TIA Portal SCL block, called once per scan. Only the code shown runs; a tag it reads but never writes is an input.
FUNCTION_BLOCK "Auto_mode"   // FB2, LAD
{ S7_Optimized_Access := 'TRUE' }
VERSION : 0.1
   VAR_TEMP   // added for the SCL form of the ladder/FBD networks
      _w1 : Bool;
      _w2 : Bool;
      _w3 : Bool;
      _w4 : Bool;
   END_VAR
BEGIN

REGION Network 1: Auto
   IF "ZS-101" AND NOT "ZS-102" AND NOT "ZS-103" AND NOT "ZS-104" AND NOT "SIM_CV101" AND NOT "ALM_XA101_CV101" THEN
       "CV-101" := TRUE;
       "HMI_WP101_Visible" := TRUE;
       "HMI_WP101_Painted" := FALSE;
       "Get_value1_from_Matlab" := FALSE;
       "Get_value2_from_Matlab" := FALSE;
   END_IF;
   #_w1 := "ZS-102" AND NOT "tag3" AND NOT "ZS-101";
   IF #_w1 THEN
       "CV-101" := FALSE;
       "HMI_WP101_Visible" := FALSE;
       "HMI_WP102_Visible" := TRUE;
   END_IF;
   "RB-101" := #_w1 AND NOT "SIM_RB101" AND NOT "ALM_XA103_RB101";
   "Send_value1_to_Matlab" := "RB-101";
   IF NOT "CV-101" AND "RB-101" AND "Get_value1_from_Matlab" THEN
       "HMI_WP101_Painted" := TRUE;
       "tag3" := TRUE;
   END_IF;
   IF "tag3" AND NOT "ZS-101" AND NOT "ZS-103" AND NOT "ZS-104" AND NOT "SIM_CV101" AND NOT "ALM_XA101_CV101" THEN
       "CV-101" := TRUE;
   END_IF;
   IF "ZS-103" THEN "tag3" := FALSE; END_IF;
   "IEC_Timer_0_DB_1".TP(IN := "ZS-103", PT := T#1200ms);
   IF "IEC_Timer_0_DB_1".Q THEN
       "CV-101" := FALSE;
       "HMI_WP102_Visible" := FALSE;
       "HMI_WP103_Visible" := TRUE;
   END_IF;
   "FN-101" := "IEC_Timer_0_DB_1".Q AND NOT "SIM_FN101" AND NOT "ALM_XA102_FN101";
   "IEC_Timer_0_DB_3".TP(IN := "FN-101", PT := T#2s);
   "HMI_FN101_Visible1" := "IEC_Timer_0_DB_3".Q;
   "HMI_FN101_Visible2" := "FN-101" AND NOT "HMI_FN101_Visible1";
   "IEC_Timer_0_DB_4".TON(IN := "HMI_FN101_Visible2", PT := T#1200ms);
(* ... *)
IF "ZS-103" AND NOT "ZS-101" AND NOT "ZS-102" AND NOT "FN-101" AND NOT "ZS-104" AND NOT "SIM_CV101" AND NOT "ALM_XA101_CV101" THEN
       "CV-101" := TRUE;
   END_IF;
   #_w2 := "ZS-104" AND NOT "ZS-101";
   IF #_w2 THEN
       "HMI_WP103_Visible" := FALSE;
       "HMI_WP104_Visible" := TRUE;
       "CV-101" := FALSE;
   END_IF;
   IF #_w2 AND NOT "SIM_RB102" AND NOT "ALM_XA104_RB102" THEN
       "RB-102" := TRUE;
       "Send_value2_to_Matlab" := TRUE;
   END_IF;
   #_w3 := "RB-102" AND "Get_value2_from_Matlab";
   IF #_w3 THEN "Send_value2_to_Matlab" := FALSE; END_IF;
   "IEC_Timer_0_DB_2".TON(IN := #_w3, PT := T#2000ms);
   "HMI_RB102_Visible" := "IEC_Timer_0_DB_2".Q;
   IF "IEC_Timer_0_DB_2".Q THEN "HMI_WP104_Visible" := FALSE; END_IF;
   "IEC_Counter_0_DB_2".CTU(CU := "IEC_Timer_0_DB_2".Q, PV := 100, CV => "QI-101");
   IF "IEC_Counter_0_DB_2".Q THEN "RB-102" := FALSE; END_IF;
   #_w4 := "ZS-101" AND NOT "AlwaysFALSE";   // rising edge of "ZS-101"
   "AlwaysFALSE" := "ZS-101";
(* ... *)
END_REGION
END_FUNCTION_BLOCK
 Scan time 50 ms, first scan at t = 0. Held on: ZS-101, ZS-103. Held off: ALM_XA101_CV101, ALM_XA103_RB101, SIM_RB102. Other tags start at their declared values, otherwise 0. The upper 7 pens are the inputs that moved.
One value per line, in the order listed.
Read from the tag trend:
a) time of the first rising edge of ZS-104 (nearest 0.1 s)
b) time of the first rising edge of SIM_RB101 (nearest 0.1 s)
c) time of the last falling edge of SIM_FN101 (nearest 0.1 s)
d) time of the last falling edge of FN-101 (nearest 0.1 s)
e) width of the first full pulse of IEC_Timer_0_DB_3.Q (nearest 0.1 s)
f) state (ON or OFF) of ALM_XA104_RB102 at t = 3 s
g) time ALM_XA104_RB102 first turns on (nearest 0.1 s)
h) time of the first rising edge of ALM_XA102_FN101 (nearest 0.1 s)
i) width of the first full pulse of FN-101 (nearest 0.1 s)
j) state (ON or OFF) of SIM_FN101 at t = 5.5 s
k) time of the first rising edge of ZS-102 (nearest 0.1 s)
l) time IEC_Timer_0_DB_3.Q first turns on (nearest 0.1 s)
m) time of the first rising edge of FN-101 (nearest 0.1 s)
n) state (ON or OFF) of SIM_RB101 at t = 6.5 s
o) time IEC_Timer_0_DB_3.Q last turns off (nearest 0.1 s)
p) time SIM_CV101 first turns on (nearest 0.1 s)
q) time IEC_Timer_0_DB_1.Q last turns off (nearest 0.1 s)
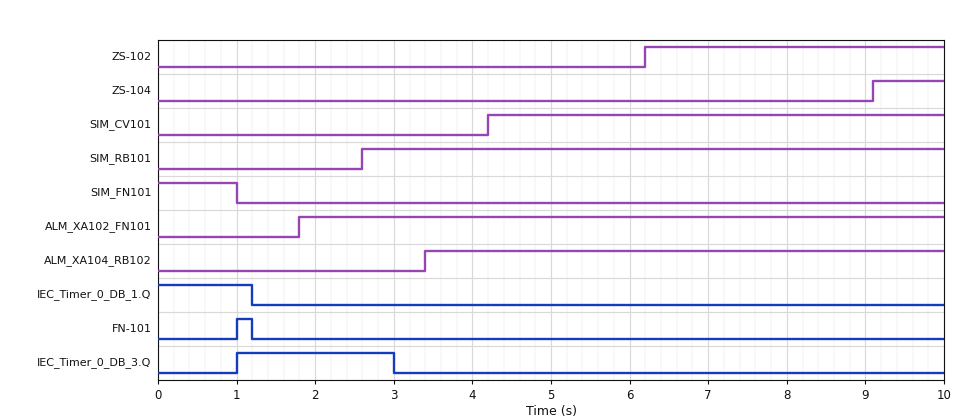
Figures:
9.1 s
2.6 s
1.0 s
1.2 s
2.0 s
OFF
3.4 s
1.8 s
0.2 s
OFF
6.2 s
1.0 s
1.0 s
ON
3.0 s
4.2 s
1.2 s
